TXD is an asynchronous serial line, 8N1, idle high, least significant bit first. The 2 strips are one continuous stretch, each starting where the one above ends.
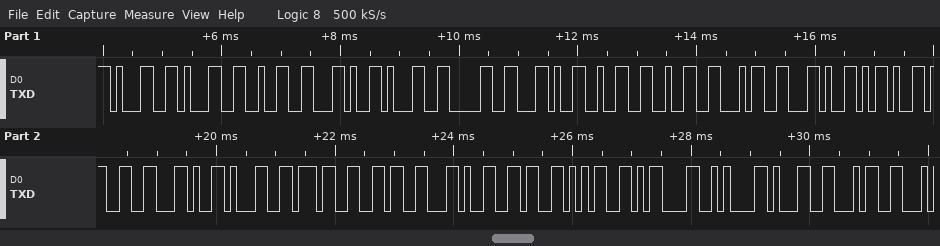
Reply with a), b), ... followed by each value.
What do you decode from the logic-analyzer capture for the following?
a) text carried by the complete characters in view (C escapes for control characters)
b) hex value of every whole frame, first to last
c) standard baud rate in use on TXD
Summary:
a) "112,10,224,-3,176,65\r\n14"
b) 31 31 32 2C 31 30 2C 32 32 34 2C 2D 33 2C 31 37 36 2C 36 35 0D 0A 31 34
c) 9600 baud
